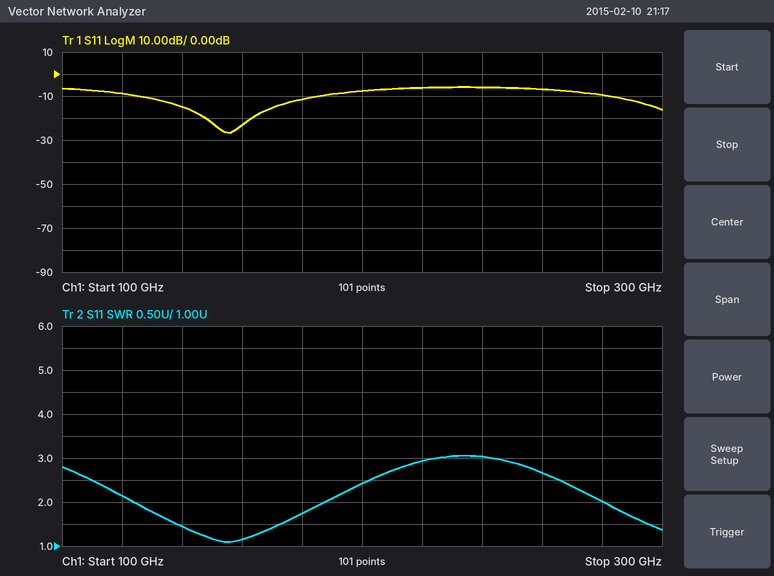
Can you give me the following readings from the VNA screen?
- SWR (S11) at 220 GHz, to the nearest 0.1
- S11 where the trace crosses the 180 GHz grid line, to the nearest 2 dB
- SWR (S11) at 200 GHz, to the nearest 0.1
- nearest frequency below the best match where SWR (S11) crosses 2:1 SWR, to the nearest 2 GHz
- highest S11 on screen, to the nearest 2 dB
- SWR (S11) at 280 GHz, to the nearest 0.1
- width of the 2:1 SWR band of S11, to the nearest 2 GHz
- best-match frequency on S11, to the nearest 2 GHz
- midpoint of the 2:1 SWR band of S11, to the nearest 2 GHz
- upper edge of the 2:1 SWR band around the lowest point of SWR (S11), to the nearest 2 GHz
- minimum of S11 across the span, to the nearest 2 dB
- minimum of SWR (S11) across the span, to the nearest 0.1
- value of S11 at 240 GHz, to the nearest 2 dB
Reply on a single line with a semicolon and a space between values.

2.9; -12 dB; 2.4; 124 GHz; -6 dB; 2.0; 64 GHz; 156 GHz; 156 GHz; 188 GHz; -26 dB; 1.1; -6 dB
